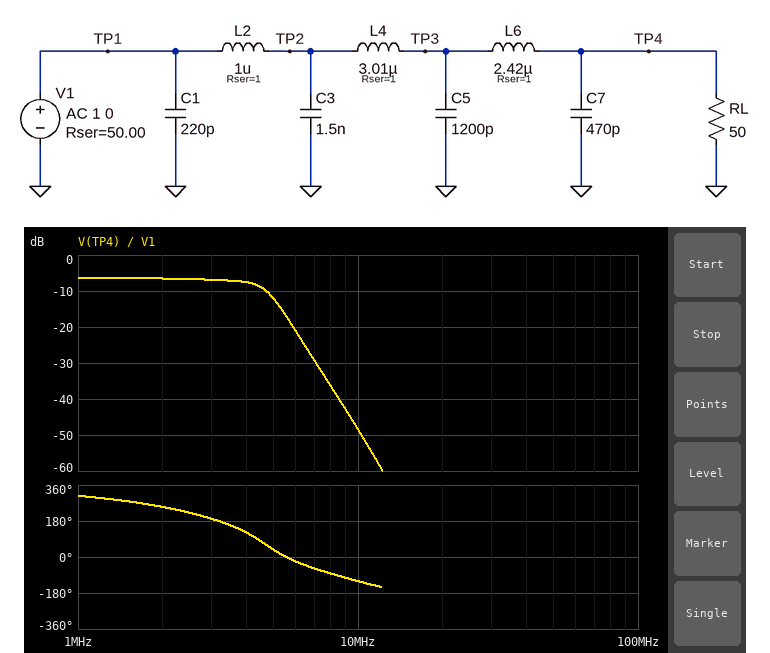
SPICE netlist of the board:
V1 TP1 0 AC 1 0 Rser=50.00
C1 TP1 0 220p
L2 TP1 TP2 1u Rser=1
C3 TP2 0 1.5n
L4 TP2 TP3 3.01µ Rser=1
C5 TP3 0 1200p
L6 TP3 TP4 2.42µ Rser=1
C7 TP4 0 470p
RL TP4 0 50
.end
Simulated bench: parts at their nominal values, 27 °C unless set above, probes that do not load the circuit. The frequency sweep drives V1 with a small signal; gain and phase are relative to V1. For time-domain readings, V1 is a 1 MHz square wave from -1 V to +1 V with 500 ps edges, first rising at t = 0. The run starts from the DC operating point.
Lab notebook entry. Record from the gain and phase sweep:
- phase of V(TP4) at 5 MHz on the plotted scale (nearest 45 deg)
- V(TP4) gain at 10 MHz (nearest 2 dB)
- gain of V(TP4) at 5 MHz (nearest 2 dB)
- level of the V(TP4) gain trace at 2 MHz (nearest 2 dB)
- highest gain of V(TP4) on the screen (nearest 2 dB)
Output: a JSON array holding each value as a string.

["45 deg", "-48 dB", "-12 dB", "-6 dB", "-6 dB"]
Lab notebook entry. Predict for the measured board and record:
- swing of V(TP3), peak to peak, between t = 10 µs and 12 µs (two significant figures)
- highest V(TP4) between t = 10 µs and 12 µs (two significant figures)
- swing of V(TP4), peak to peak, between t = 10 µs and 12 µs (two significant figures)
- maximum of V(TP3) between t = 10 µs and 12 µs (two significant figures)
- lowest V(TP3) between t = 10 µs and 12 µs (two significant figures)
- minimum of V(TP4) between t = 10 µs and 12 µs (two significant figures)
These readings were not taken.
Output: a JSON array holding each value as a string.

["1.3 V", "600 mV", "1.2 V", "640 mV", "-640 mV", "-600 mV"]
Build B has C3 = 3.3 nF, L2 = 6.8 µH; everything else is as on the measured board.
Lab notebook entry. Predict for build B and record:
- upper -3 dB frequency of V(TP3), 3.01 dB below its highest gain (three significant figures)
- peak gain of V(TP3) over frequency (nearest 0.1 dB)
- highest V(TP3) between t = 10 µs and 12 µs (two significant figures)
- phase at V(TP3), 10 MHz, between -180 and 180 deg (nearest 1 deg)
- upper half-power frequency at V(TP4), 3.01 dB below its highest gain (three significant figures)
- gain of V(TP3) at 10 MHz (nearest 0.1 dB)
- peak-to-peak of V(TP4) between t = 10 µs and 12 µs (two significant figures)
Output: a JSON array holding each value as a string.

["1.74 MHz", "-6.1 dB", "540 mV", "-28 deg", "1.72 MHz", "-61.3 dB", "1.1 V"]
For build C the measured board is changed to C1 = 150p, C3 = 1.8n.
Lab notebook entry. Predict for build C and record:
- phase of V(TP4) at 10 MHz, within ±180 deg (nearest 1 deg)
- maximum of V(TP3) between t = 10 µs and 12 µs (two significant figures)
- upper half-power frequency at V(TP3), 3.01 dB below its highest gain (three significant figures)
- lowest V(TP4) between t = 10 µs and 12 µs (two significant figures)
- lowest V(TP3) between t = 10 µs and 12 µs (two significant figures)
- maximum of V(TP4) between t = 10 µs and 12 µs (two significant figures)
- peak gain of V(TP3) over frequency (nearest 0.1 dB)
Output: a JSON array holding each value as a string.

["-112 deg", "610 mV", "4.84 MHz", "-580 mV", "-610 mV", "580 mV", "-6.1 dB"]
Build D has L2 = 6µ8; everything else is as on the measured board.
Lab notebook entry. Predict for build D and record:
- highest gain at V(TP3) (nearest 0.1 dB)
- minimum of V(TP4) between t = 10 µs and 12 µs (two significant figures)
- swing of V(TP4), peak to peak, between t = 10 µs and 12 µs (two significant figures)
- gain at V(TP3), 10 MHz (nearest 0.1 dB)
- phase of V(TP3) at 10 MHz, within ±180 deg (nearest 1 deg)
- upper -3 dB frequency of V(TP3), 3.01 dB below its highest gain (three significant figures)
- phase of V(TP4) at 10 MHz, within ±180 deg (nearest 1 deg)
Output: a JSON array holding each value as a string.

["-6.1 dB", "-530 mV", "1.1 V", "-54.0 dB", "-28 deg", "2.96 MHz", "-167 deg"]
